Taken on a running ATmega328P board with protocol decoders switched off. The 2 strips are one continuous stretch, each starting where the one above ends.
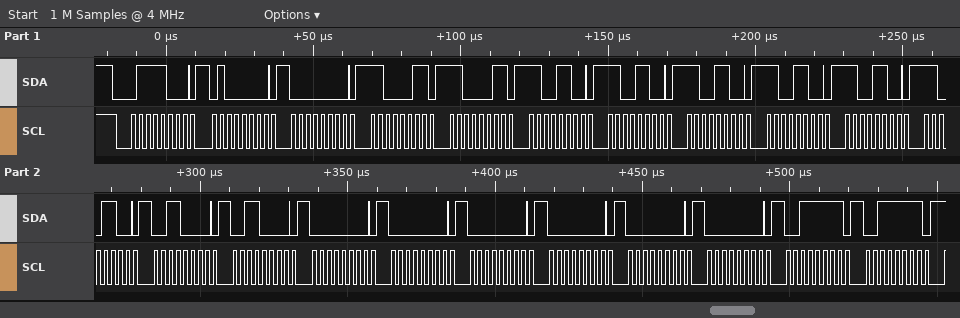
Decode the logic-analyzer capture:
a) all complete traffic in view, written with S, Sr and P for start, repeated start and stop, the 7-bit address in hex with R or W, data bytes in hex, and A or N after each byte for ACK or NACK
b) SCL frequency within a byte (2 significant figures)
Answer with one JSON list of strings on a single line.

["S 3CW A 40 A 00 A C3 A C3 A CC A CC A CC A CC A CC A CC A 30 A 30 A 00 A 00 A 00 A 00 A 00 A 00 A 3F A 3F A", "400 kHz"]
